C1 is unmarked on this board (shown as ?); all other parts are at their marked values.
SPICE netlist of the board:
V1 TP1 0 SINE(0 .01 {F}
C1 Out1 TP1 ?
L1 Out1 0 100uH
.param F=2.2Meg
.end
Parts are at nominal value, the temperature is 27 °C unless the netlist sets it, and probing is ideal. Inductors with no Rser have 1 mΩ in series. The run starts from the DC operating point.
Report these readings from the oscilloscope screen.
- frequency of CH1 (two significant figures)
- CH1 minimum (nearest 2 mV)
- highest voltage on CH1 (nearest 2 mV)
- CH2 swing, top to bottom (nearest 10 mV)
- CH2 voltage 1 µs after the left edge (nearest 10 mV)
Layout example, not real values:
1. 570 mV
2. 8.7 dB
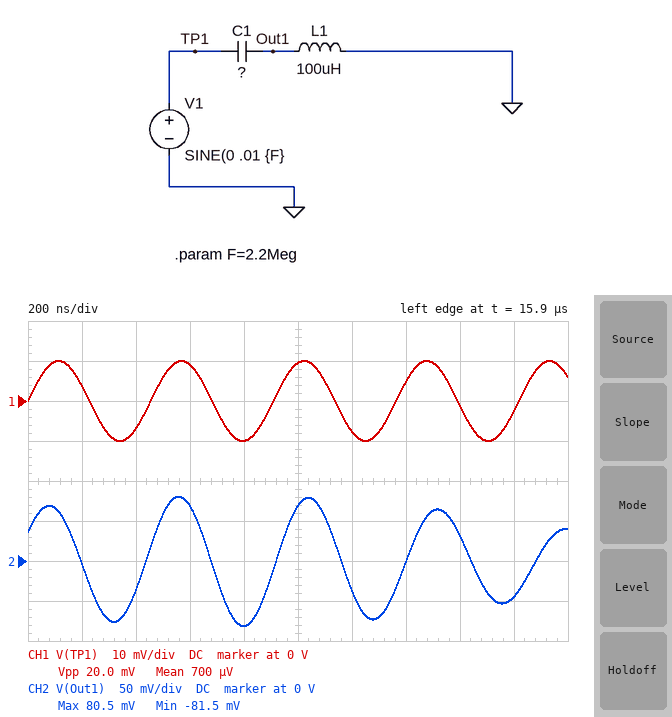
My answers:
1. 2.2 MHz
2. -10 mV
3. 10 mV
4. 160 mV
5. 70 mV
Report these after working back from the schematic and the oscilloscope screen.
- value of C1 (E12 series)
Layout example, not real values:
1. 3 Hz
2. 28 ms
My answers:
1. 68 pF
